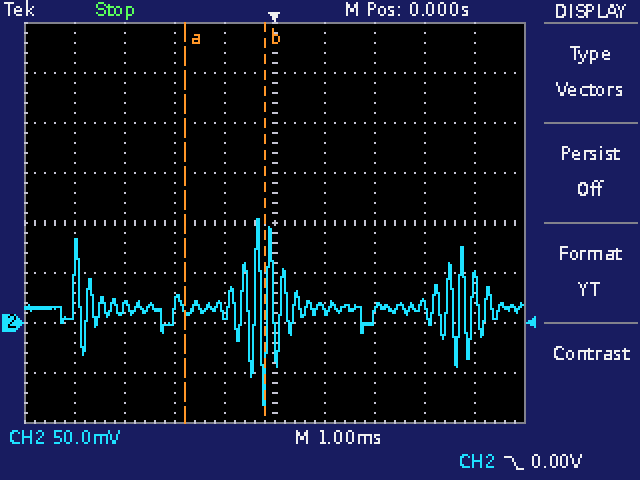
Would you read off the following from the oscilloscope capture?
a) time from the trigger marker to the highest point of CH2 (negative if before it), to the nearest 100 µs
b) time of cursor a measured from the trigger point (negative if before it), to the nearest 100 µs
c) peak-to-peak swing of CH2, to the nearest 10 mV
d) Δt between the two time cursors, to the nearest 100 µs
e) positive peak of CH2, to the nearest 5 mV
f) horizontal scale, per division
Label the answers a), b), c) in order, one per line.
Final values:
a) -300 µs
b) -1.8 ms
c) 190 mV
d) 1.6 ms
e) 105 mV
f) 1 ms
